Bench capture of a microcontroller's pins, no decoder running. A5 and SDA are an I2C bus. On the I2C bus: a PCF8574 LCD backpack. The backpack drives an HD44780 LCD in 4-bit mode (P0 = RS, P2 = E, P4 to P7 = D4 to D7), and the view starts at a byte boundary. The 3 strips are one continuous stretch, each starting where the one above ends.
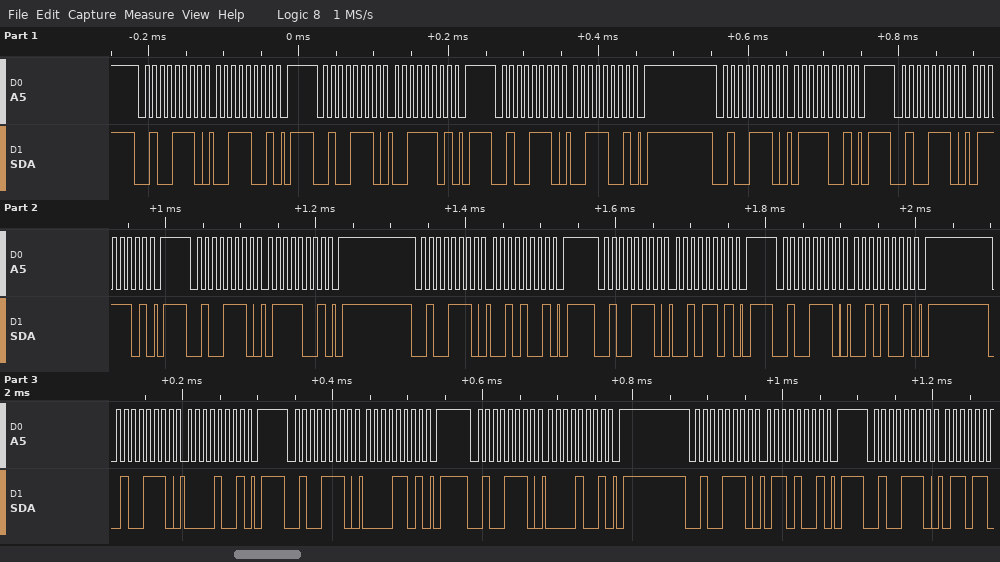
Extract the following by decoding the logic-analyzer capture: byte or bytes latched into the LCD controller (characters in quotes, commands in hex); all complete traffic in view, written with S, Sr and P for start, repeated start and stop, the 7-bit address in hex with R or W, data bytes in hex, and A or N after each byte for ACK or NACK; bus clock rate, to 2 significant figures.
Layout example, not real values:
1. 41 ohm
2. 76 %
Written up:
1. '7' ' '
2. S 27W A 39 A P S 27W A 3D A P S 27W A 39 A P S 27W A 79 A P S 27W A 7D A P S 27W A 79 A P S 27W A 29 A P S 27W A 2D A P S 27W A 29 A P S 27W A 09 A P S 27W A 0D A P S 27W A 09 A P S 27W A 69 A P S 27W A
3. 100 kHz
